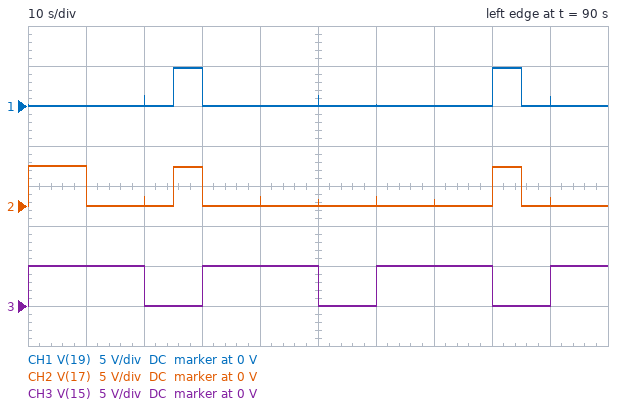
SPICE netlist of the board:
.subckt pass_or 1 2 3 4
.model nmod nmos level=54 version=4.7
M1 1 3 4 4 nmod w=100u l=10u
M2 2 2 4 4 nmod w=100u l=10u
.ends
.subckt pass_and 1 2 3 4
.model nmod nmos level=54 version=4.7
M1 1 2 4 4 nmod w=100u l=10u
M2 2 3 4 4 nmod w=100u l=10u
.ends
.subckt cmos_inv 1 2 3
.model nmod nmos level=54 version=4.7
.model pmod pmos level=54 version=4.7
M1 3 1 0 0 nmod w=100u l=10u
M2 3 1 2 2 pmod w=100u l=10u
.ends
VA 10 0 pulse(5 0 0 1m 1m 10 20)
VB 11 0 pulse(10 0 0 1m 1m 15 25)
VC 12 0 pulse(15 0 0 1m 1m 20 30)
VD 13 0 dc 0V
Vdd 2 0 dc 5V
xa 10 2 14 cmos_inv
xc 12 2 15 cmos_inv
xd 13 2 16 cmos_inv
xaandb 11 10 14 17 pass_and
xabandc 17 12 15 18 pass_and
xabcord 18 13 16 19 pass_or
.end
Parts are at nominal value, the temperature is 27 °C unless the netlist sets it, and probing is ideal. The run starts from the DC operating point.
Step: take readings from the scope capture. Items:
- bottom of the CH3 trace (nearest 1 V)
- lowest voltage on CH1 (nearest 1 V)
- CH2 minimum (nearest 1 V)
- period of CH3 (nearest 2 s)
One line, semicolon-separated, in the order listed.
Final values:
0 V; 0 V; 0 V; 30 s
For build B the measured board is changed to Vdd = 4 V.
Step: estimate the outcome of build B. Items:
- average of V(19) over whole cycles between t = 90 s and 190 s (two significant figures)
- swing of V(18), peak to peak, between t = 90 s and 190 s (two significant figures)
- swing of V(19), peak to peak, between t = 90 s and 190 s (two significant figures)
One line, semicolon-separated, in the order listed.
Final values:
350 mV; 4.8 V; 3.8 V
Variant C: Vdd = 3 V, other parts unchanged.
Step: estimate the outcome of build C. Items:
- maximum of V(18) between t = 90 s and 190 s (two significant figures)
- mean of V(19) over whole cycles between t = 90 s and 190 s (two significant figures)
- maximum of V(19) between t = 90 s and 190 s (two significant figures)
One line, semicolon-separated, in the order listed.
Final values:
4.8 V; 260 mV; 2.8 V
